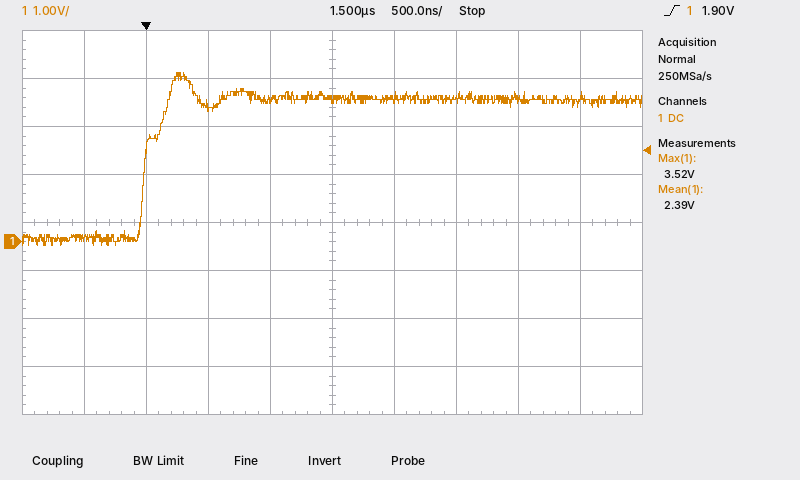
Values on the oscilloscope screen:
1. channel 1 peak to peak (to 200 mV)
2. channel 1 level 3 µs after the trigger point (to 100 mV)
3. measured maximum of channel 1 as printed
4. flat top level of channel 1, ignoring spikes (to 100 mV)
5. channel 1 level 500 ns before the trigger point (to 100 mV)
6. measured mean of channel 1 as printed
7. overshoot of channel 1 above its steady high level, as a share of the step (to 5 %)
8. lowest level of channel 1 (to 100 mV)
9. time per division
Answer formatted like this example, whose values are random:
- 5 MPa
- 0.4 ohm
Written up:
- 3.6 V
- 3.0 V
- 3.52 V
- 3.0 V
- 100 mV
- 2.39 V
- 20 %
- -100 mV
- 500 ns
